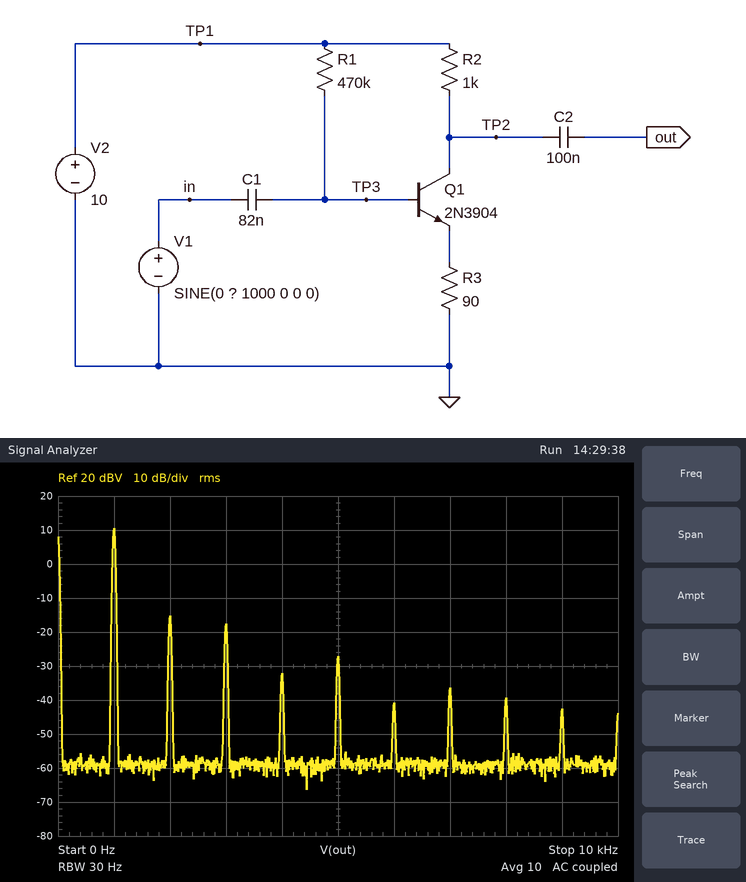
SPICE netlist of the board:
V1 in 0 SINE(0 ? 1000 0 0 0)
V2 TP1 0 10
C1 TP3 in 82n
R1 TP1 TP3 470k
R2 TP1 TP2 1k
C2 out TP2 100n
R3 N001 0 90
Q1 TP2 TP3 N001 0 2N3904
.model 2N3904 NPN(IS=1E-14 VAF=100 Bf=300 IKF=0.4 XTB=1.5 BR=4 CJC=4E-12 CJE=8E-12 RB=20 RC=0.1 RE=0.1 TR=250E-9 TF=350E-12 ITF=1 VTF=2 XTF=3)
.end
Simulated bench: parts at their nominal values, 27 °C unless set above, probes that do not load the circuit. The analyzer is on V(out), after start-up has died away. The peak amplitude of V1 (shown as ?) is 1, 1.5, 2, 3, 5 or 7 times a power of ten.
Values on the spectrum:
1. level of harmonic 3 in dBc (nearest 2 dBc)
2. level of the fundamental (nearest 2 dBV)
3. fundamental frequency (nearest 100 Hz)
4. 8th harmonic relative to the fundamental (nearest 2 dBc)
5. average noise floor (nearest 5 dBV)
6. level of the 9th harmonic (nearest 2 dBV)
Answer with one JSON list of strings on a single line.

["-28 dBc", "10 dBV", "1.0 kHz", "-50 dBc", "-60 dBV", "-42 dBV"]
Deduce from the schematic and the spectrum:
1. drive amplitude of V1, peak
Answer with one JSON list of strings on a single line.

["500 mV"]
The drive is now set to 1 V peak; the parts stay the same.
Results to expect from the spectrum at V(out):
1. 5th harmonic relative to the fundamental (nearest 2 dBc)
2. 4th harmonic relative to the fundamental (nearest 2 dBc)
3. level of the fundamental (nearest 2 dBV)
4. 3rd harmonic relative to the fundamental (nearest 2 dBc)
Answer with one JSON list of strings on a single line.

["-30 dBc", "-20 dBc", "10 dBV", "-32 dBc"]
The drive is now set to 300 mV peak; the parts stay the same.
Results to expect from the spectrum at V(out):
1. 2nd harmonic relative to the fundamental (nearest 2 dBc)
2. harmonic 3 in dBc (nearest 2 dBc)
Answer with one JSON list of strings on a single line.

["-42 dBc", "-56 dBc"]
